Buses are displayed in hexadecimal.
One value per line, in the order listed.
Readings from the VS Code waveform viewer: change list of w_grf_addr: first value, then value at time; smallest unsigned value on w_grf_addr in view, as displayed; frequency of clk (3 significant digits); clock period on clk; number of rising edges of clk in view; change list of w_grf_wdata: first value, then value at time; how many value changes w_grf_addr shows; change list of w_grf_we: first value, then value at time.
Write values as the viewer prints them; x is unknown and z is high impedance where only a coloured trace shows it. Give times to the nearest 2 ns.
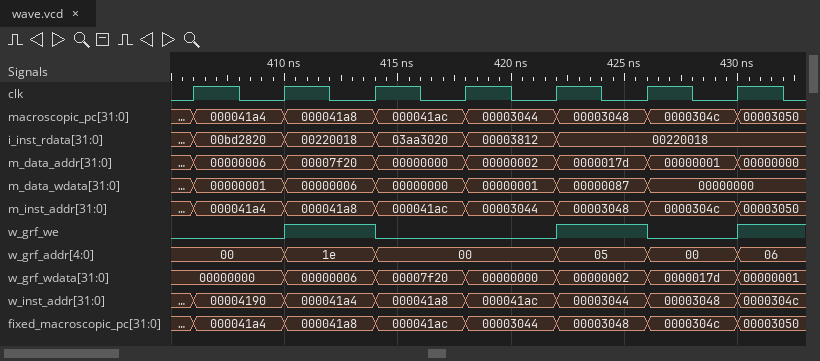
00, 1e at 410 ns, 00 at 414 ns, 05 at 422 ns, 00 at 426 ns, 06 at 430 ns
00
250 MHz
4 ns
7
00000000, 00000006 at 410 ns, 00007f20 at 414 ns, 00000000 at 418 ns, 00000002 at 422 ns, 0000017d at 426 ns, 00000001 at 430 ns
5
0, 1 at 410 ns, 0 at 414 ns, 1 at 422 ns, 0 at 426 ns, 1 at 430 ns
